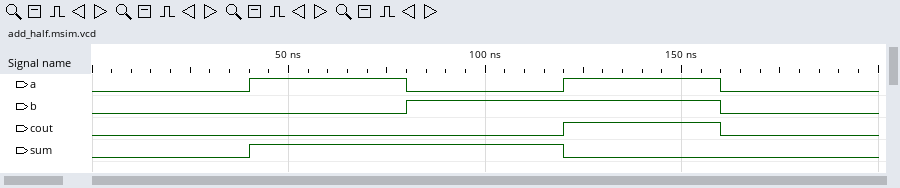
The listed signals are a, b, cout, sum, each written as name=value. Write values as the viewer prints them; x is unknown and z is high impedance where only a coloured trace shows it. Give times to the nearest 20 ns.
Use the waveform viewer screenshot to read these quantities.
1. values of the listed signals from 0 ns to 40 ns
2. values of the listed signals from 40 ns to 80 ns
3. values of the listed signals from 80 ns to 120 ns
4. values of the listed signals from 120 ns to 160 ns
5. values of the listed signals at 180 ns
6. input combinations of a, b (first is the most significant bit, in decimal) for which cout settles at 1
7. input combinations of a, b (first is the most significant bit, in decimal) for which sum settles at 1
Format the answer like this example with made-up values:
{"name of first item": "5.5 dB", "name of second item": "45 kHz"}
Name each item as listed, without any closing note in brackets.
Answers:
{"values of the listed signals from 0 ns to 40 ns": "a=0, b=0, cout=0, sum=0", "values of the listed signals from 40 ns to 80 ns": "a=1, b=0, cout=0, sum=1", "values of the listed signals from 80 ns to 120 ns": "a=0, b=1, cout=0, sum=1", "values of the listed signals from 120 ns to 160 ns": "a=1, b=1, cout=1, sum=0", "values of the listed signals at 180 ns": "a=0, b=0, cout=0, sum=0", "input combinations of a, b (first is the most significant bit, in decimal) for which cout settles at 1": "3", "input combinations of a, b (first is the most significant bit, in decimal) for which sum settles at 1": "1, 2"}
